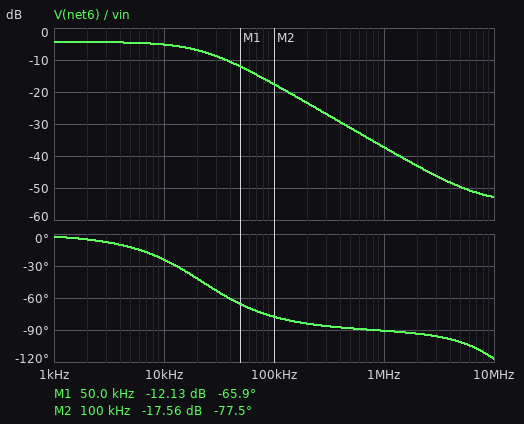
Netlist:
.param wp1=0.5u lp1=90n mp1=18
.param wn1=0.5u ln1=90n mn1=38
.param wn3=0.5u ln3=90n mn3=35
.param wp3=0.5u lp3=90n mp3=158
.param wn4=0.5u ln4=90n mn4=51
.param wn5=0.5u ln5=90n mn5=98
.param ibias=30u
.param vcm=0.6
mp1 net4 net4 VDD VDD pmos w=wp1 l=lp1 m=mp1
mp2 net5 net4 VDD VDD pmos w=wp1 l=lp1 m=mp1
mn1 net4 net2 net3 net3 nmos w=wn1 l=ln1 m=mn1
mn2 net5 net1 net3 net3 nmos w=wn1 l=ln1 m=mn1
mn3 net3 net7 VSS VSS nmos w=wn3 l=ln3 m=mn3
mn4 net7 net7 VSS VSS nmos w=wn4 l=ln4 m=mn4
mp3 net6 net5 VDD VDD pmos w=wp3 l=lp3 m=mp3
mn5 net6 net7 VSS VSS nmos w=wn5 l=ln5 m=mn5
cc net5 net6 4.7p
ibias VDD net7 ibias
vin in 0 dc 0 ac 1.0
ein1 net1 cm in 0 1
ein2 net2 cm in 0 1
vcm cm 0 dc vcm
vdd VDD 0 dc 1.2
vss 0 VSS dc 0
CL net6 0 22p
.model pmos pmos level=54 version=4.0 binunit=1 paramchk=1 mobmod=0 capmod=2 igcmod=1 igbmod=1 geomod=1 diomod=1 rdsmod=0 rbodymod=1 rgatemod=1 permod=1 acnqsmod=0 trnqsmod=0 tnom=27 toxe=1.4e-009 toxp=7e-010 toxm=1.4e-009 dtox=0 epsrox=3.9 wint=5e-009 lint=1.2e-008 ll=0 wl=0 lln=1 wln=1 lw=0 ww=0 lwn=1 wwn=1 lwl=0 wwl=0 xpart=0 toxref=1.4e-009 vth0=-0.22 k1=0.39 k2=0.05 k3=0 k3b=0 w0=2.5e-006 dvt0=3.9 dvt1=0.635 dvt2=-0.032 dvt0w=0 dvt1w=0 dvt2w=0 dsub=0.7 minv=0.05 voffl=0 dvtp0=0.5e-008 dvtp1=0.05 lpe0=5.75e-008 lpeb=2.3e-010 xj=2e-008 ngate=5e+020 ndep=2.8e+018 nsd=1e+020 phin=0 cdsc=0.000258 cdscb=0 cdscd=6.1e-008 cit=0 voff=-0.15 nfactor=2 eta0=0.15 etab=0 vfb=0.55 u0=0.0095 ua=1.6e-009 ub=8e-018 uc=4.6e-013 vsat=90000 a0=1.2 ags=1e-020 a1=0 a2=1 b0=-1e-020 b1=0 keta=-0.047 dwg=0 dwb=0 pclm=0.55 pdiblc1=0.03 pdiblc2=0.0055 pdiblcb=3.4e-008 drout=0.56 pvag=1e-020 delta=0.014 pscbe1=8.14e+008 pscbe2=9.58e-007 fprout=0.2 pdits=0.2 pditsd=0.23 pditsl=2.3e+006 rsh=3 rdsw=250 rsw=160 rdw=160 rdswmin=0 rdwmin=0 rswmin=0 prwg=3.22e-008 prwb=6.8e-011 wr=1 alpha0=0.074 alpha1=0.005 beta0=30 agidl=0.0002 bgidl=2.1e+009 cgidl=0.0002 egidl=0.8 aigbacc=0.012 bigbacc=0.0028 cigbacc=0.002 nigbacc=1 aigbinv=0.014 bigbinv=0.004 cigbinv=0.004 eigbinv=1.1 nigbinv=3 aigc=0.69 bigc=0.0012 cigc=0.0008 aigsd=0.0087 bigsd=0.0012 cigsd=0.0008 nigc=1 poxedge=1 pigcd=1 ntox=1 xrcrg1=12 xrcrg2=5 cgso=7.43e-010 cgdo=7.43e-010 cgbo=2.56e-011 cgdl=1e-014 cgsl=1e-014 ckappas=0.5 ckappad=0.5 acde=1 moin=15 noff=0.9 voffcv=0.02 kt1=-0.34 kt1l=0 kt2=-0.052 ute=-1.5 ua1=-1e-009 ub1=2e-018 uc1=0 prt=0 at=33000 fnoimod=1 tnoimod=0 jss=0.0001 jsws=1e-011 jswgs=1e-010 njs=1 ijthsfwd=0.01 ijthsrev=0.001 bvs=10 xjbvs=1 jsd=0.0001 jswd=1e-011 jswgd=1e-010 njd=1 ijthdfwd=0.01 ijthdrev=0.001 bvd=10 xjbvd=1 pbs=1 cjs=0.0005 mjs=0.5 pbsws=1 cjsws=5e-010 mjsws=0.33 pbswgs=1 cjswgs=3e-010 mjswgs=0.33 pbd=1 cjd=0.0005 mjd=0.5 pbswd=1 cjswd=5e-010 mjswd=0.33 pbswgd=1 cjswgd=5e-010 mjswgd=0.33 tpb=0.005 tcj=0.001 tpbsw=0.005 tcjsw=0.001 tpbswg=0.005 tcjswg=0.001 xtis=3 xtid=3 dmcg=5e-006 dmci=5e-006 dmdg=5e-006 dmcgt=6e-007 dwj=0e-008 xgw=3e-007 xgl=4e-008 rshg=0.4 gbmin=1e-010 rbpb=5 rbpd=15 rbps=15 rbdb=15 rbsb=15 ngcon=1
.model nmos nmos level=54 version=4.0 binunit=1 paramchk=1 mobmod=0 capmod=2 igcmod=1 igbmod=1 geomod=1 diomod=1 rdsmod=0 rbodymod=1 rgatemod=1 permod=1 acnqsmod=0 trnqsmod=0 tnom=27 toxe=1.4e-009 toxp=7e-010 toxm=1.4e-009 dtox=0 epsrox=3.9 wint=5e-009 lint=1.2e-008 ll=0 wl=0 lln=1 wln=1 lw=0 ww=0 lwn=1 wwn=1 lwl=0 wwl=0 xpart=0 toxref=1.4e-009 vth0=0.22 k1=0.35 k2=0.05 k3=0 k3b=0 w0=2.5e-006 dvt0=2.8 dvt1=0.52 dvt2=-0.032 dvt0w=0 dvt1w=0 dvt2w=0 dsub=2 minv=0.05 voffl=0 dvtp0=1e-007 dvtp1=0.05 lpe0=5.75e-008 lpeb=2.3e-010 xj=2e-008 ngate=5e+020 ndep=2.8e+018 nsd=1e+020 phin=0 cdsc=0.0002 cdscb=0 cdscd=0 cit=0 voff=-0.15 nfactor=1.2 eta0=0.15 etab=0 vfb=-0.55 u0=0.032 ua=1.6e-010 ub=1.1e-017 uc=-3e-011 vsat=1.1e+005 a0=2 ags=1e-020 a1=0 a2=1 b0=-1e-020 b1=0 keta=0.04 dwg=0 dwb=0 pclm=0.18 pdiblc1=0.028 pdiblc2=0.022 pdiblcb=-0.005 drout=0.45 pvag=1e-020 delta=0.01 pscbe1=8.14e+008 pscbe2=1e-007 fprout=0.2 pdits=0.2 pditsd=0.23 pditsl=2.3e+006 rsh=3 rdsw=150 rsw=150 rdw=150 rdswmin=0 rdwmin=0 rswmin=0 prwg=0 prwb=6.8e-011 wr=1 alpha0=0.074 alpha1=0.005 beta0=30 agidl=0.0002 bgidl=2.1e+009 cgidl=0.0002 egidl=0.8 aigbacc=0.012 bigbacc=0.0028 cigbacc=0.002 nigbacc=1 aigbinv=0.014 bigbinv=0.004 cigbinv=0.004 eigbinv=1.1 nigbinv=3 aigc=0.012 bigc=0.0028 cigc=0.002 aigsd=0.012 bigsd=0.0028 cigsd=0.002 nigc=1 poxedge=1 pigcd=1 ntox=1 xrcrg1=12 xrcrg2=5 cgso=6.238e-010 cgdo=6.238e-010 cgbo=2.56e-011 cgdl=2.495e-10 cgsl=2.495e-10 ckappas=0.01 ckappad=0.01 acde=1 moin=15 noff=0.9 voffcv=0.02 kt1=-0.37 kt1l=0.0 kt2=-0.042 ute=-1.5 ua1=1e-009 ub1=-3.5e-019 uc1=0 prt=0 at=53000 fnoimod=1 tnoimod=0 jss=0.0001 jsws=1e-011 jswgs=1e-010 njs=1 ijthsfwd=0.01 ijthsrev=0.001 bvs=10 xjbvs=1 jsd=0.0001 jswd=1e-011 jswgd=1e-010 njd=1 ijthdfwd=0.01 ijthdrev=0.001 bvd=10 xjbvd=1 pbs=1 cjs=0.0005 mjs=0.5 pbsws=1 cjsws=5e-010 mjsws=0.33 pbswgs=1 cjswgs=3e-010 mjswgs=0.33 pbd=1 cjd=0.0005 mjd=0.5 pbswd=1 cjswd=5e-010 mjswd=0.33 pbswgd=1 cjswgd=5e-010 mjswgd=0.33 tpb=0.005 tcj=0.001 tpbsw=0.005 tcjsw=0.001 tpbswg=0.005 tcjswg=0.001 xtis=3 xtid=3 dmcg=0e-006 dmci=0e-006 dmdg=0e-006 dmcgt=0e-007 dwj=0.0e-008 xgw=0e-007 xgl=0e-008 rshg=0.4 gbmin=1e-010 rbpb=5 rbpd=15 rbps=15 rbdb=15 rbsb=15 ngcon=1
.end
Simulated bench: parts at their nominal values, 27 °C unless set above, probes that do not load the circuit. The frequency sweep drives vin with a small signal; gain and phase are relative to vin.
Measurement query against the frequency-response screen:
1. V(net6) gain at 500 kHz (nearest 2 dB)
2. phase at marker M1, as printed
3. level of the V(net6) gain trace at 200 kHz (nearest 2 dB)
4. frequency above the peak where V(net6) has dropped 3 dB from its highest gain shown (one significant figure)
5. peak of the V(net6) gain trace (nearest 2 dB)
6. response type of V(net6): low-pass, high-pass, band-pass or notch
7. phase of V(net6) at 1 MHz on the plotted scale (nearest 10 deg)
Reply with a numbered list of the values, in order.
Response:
1. -32 dB
2. -65.9 deg
3. -24 dB
4. 20 kHz
5. -4 dB
6. low-pass
7. -90 deg
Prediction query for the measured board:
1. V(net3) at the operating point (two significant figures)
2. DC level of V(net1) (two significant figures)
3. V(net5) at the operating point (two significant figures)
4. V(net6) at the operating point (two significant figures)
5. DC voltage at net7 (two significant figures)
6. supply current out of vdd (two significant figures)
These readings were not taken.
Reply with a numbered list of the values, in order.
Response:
1. 340 mV
2. 600 mV
3. 870 mV
4. 940 mV
5. 300 mV
6. 140 µA
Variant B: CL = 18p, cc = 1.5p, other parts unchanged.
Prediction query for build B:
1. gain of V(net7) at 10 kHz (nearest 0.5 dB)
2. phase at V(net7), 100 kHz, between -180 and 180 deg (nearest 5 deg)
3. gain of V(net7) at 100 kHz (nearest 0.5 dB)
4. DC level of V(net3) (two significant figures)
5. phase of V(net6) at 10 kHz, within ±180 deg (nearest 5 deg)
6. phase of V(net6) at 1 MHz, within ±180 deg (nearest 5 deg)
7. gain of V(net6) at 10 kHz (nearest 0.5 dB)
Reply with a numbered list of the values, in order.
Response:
1. -41.5 dB
2. -55 deg
3. -46.5 dB
4. 340 mV
5. -10 deg
6. -85 deg
7. -4.5 dB
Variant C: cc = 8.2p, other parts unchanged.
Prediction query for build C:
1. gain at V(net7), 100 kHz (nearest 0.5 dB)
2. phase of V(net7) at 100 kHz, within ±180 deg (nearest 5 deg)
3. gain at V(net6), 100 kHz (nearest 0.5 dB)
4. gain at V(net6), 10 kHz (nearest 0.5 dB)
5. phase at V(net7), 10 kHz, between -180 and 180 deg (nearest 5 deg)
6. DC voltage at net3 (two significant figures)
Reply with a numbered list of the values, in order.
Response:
1. -59.0 dB
2. -80 deg
3. -22.0 dB
4. -6.5 dB
5. -35 deg
6. 340 mV
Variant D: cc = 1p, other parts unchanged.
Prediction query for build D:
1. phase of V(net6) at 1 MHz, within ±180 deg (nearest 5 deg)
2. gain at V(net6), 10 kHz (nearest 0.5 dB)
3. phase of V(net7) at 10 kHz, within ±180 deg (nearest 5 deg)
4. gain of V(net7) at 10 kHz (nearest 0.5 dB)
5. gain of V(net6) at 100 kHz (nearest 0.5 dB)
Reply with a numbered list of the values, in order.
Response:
1. -85 deg
2. -4.5 dB
3. -5 deg
4. -41.5 dB
5. -8.0 dB
